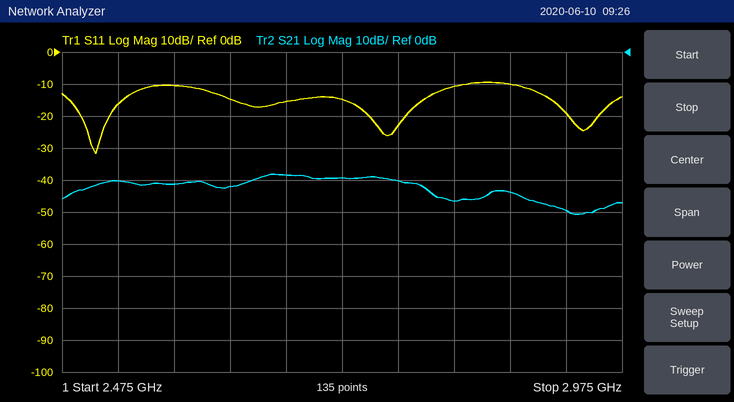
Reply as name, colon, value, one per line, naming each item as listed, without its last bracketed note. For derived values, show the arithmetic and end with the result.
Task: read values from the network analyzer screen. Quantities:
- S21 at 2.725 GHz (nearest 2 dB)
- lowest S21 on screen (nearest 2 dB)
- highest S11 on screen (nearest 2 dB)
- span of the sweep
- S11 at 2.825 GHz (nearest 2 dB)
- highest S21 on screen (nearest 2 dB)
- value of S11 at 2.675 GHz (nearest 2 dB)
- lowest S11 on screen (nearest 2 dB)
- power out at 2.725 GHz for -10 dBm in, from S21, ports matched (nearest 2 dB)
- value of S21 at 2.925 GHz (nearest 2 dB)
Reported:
S21 at 2.725 GHz: -40 dB
lowest S21 on screen: -50 dB
highest S11 on screen: -10 dB
span of the sweep: 500 MHz
S11 at 2.825 GHz: -10 dB
highest S21 on screen: -38 dB
value of S11 at 2.675 GHz: -16 dB
lowest S11 on screen: -32 dB
power out at 2.725 GHz for -10 dBm in, from S21, ports matched: -10 dBm + (-40 dB) = -50 dBm
value of S21 at 2.925 GHz: -50 dB
